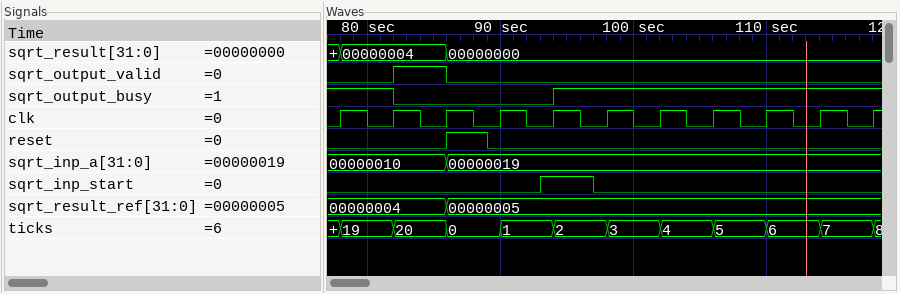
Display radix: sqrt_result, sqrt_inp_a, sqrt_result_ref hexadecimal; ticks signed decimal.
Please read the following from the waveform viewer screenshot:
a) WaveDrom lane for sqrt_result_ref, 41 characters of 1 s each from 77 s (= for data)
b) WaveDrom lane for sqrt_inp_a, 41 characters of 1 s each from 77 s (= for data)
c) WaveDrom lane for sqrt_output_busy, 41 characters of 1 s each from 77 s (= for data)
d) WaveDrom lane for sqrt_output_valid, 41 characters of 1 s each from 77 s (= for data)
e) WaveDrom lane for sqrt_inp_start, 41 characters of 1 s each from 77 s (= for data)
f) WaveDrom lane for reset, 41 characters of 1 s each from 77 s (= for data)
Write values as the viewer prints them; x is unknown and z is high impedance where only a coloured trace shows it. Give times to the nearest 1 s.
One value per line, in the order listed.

{name: 'sqrt_result_ref', wave: '=........=...............................', data: '00000004 00000005'}
{name: 'sqrt_inp_a', wave: '=........=...............................', data: '00000010 00000019'}
{name: 'sqrt_output_busy', wave: '1....0...........1.......................'}
{name: 'sqrt_output_valid', wave: '0....1...0...............................'}
{name: 'sqrt_inp_start', wave: '0...............1...0....................'}
{name: 'reset', wave: '0........1..0............................'}
